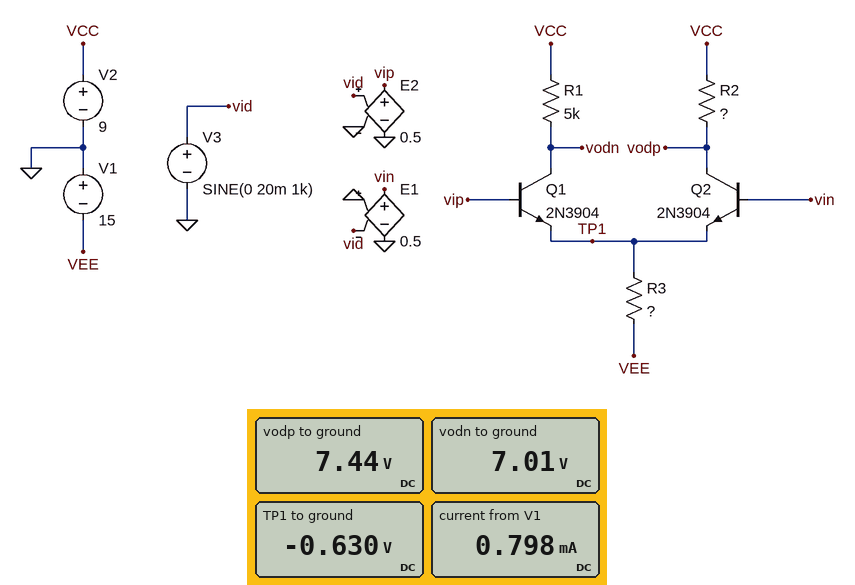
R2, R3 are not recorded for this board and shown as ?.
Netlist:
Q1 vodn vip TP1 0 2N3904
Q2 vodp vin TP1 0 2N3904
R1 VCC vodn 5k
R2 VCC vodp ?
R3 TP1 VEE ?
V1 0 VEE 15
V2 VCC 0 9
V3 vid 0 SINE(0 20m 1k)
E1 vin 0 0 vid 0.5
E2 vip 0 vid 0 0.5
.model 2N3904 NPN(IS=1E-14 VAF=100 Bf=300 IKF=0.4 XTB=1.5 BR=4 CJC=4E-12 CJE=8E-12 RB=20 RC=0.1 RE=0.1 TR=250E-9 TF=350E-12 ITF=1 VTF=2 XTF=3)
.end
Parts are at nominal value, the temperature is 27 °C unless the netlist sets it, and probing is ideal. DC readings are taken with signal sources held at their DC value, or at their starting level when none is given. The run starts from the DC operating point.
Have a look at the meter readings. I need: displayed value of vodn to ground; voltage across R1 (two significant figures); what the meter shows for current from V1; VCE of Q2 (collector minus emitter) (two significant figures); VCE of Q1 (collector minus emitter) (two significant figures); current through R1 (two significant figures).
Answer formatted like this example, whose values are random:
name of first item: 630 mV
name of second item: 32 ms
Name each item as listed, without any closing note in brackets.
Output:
displayed value of vodn to ground: 7.01 V
voltage across R1: 2.0 V
what the meter shows for current from V1: 0.798 mA
VCE of Q2 (collector minus emitter): 8.1 V
VCE of Q1 (collector minus emitter): 7.6 V
current through R1: 400 µA
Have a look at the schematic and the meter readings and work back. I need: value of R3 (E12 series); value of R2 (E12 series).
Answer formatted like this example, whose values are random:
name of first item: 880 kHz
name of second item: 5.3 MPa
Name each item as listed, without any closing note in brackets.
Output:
value of R3: 18 kΩ
value of R2: 3.9 kΩ
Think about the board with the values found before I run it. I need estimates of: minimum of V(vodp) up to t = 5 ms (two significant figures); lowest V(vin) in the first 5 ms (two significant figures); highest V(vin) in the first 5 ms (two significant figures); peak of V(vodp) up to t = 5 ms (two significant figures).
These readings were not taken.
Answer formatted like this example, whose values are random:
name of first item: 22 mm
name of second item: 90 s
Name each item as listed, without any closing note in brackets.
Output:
minimum of V(vodp) up to t = 5 ms: 6.9 V
lowest V(vin) in the first 5 ms: -10 mV
highest V(vin) in the first 5 ms: 10 mV
peak of V(vodp) up to t = 5 ms: 8.0 V
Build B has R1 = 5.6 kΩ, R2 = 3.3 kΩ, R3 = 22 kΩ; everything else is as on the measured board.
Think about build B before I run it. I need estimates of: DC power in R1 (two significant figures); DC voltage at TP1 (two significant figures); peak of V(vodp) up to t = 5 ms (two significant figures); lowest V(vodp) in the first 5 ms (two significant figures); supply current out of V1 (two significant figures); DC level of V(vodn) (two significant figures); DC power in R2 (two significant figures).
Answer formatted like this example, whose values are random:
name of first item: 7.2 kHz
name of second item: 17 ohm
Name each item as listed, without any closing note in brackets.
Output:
DC power in R1: 590 µW
DC voltage at TP1: -620 mV
peak of V(vodp) up to t = 5 ms: 8.3 V
lowest V(vodp) in the first 5 ms: 7.5 V
supply current out of V1: 650 µA
DC level of V(vodn): 7.2 V
DC power in R2: 350 µW
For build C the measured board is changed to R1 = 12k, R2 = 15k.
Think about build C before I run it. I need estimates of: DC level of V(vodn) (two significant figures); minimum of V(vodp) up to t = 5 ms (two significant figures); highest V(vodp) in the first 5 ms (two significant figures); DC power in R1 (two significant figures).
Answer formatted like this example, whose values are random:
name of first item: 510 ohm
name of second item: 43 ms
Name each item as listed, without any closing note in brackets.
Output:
DC level of V(vodn): 4.2 V
minimum of V(vodp) up to t = 5 ms: 960 mV
highest V(vodp) in the first 5 ms: 5.2 V
DC power in R1: 1.9 mW
